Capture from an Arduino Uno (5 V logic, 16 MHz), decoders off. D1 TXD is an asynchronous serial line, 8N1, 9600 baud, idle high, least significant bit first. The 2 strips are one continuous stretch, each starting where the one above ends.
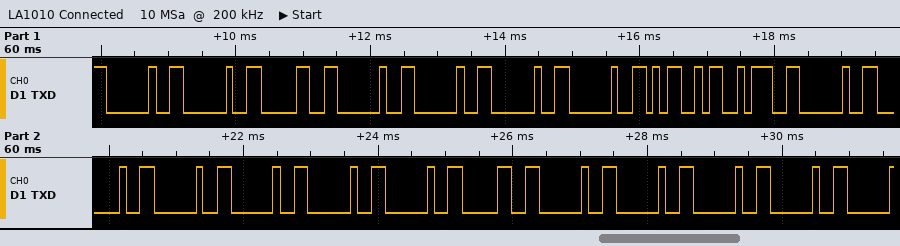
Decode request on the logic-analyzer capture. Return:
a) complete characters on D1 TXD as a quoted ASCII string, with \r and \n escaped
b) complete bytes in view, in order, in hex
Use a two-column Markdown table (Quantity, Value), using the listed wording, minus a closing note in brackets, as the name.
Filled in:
| Quantity | Value |
|---|---|
| complete characters on D1 TXD as a quoted ASCII string, with \r and \n escaped | "  0    M:      0    " |
| complete bytes in view, in order, in hex | 20 20 30 20 20 20 20 4D 3A 20 20 20 20 20 20 30 20 20 20 20 |
